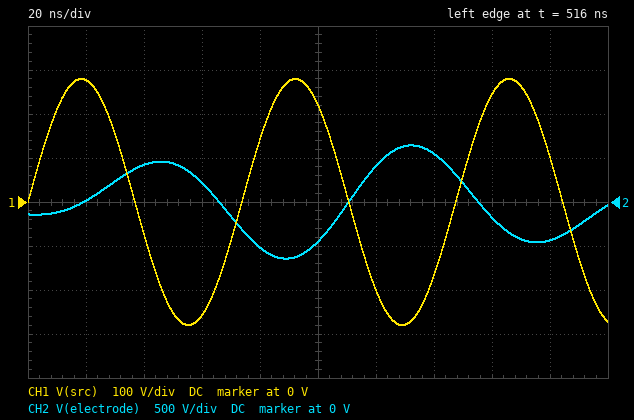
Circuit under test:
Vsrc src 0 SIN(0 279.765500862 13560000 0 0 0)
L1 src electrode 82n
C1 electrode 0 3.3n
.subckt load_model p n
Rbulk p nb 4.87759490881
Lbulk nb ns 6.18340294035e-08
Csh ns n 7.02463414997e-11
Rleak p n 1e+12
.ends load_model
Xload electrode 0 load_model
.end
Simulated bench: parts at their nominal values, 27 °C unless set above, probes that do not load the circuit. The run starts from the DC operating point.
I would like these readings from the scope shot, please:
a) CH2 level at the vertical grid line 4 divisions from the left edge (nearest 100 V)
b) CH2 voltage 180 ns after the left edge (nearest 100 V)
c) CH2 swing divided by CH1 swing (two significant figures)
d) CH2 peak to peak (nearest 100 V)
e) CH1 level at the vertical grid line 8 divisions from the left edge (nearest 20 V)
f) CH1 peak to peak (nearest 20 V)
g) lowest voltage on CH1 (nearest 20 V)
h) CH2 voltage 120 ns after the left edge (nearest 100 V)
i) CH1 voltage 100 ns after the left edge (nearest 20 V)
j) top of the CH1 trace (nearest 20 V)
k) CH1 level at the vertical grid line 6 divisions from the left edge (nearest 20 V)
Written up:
-500 V
-400 V
2.3
1.3 kV
240 V
560 V
-280 V
400 V
220 V
280 V
-200 V
